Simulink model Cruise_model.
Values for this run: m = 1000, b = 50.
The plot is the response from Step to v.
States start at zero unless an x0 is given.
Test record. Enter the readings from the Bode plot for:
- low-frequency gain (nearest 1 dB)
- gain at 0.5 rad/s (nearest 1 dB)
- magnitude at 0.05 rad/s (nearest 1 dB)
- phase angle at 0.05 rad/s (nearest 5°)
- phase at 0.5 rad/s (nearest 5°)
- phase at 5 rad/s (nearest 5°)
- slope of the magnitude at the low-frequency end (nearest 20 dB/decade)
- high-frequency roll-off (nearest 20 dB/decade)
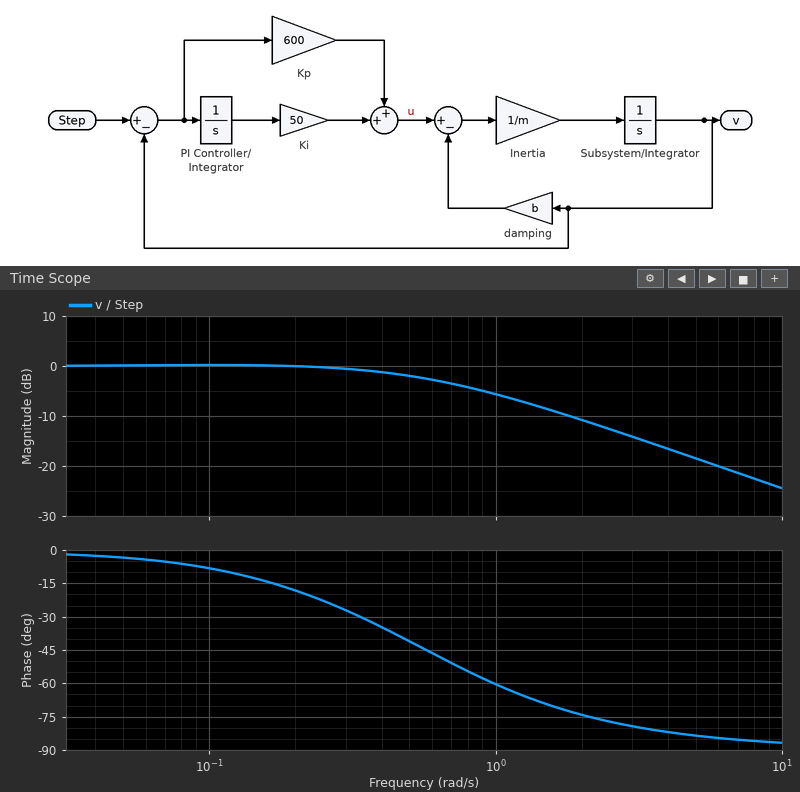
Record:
0 dB
-2 dB
0 dB
-5°
-40°
-85°
0 dB/decade
-20 dB/decade
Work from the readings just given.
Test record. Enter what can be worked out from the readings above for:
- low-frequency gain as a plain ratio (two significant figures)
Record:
1.0
